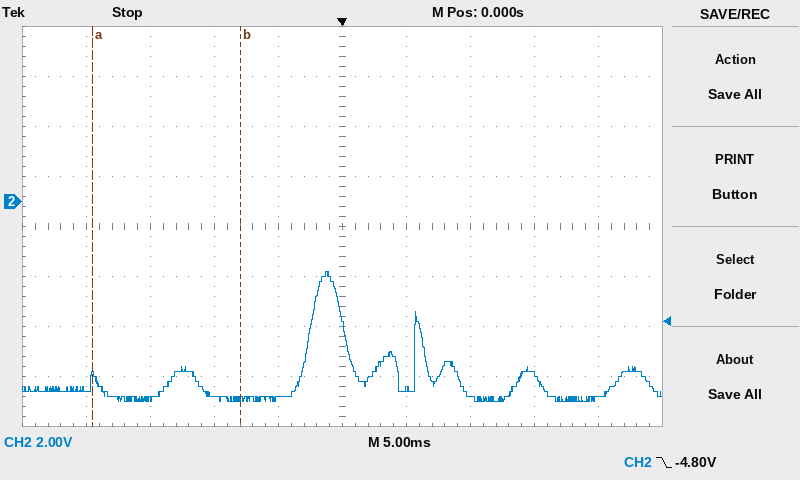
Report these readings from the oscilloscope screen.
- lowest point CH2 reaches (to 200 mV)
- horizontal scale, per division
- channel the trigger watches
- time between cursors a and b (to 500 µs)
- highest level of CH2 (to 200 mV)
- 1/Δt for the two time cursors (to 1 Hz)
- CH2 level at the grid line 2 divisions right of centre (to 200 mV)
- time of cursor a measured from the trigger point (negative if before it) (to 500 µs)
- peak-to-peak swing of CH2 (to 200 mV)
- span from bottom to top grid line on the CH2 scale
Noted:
-8.0 V
5 ms
CH2
11.5 ms
-2.8 V
87 Hz
-7.8 V
-19.5 ms
5.2 V
16 V
